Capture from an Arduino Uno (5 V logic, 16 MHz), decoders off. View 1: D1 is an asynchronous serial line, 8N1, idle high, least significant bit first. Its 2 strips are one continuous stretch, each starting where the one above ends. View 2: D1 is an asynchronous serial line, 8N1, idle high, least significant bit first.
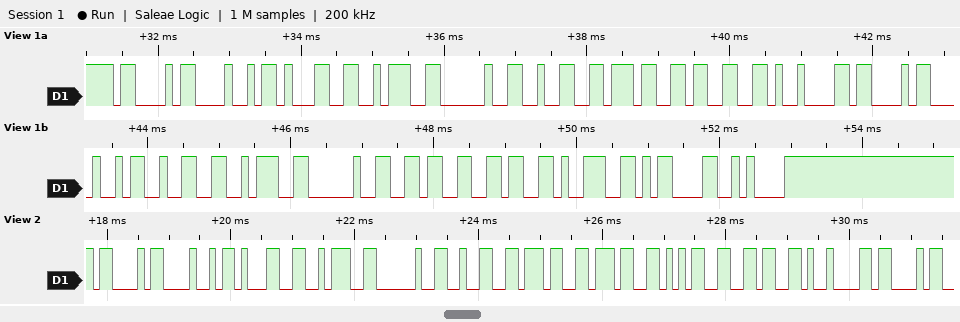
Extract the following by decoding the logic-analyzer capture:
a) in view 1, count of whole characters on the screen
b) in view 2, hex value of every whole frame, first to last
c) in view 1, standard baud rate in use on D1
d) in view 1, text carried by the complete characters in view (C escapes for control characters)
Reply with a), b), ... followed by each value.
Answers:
a) 19
b) 43 48 31 3A 20 32 37 37 35 36 09 43
c) 9600 baud
d) "CH1: 273\tCH2: 669\r\n"
